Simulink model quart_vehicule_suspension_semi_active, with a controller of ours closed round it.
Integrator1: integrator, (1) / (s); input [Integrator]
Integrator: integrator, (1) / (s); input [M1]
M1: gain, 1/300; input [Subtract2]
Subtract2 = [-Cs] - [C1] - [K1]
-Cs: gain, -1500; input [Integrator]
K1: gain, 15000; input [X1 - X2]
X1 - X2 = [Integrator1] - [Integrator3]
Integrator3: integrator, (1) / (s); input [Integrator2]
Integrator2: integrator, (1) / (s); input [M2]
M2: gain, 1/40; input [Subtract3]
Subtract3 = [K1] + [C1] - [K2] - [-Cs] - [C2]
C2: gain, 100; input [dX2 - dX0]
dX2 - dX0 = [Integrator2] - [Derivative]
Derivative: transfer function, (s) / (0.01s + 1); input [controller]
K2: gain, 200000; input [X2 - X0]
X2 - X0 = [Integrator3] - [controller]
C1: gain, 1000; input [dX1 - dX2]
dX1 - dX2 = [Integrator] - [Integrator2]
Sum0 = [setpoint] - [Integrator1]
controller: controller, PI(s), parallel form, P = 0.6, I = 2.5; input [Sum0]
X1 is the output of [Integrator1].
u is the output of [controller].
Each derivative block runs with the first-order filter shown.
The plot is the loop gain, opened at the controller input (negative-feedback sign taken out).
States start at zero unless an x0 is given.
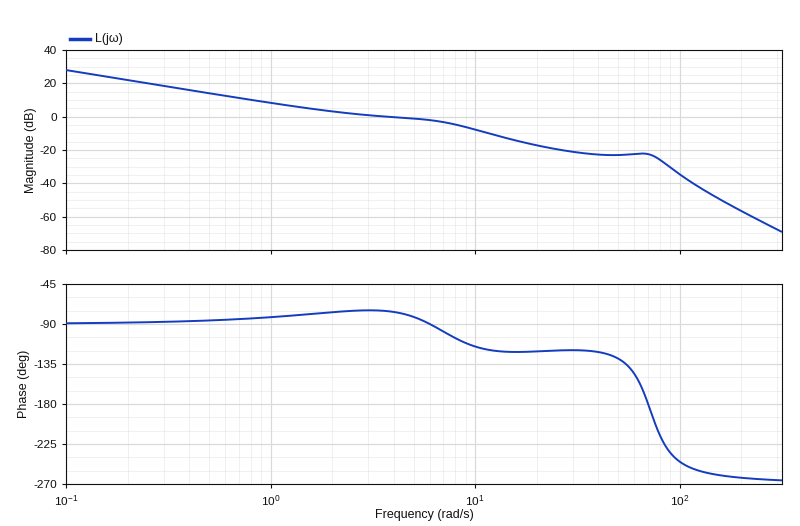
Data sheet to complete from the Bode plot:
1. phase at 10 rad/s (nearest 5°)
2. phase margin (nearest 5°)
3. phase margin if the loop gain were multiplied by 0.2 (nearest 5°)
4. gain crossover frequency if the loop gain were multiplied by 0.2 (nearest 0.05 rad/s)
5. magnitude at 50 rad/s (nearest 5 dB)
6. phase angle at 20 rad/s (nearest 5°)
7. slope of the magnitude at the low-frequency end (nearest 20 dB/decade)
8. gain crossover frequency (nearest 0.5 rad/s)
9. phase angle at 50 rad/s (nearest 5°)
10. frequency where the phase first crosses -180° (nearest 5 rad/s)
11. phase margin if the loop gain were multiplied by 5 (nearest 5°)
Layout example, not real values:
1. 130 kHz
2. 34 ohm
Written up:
1. -115°
2. 105°
3. 95°
4. 0.50 rad/s
5. -25 dB
6. -120°
7. -20 dB/decade
8. 3.5 rad/s
9. -130°
10. 70 rad/s
11. 60°
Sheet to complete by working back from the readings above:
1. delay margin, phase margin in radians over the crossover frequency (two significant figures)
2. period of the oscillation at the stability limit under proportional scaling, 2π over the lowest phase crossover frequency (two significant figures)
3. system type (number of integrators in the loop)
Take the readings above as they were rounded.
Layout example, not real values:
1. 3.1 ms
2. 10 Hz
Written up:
1. 0.52 s
2. 0.090 s
3. 1
